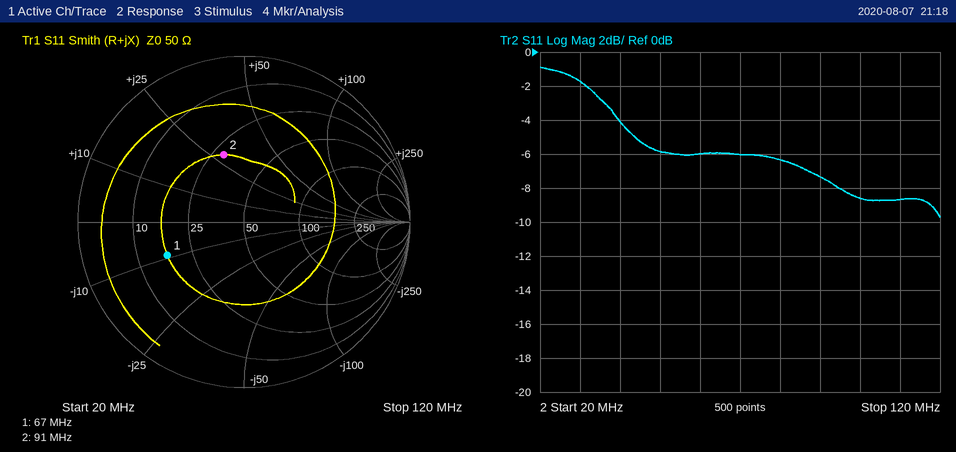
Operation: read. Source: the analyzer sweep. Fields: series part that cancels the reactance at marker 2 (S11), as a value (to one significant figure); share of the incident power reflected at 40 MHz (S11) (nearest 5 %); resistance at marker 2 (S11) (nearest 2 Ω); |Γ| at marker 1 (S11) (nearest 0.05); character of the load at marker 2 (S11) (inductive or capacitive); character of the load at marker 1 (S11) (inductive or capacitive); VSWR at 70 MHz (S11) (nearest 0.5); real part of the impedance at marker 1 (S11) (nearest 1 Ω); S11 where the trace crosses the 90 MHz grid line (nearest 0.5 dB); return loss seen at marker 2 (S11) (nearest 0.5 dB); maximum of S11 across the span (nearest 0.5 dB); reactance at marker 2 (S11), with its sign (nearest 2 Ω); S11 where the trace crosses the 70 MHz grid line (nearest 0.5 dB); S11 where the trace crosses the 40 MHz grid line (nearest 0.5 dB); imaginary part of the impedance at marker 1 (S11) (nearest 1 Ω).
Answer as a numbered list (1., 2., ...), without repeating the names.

1. 60 pF
2. 40 %
3. 28 Ω
4. 0.50
5. inductive
6. capacitive
7. 3.0
8. 17 Ω
9. -7.5 dB
10. 7.5 dB
11. -1.0 dB
12. +28 Ω
13. -6.0 dB
14. -4.0 dB
15. -9 Ω
